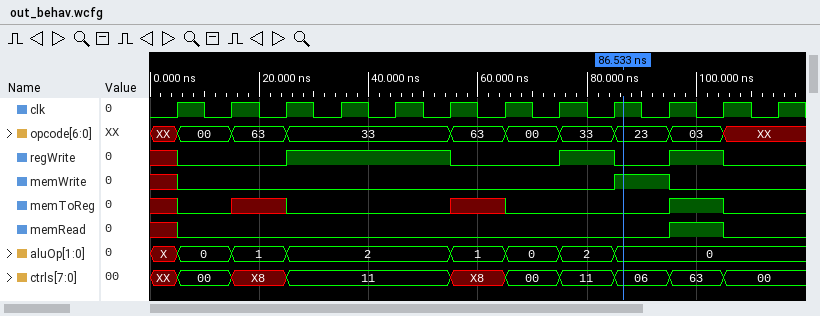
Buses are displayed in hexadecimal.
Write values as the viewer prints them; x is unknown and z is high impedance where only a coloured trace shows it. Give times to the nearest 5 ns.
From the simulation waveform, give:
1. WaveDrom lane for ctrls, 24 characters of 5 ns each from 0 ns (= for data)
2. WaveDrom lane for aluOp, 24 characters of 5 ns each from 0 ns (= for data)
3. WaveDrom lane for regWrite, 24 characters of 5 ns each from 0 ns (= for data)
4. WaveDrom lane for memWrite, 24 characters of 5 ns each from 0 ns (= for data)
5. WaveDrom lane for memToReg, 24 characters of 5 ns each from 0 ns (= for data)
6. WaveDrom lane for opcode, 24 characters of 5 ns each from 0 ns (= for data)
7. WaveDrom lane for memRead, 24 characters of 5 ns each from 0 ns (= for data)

{name: 'ctrls', wave: 'x=.=.=.....=.=.=.=.=.=..', data: '00 X8 11 X8 00 11 06 63 00'}
{name: 'aluOp', wave: 'x=.=.=.....=.=.=.=......', data: '0 1 2 1 0 2 0'}
{name: 'regWrite', wave: 'x0...1.....0...1.0.1.0..'}
{name: 'memWrite', wave: 'x0...............1.0....'}
{name: 'memToReg', wave: 'x0.x.0.....x.0.....1.0..'}
{name: 'opcode', wave: 'x=.=.=.....=.=.=.=.=.x..', data: '00 63 33 63 00 33 23 03'}
{name: 'memRead', wave: 'x0.................1.0..'}
